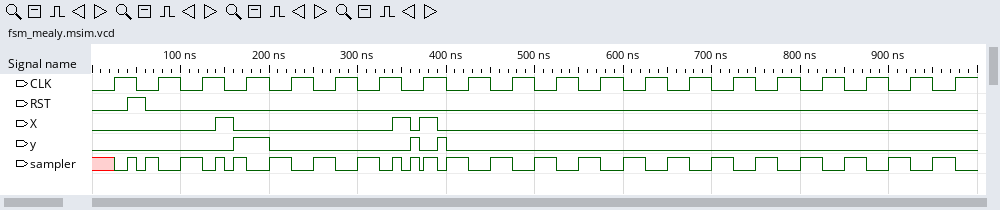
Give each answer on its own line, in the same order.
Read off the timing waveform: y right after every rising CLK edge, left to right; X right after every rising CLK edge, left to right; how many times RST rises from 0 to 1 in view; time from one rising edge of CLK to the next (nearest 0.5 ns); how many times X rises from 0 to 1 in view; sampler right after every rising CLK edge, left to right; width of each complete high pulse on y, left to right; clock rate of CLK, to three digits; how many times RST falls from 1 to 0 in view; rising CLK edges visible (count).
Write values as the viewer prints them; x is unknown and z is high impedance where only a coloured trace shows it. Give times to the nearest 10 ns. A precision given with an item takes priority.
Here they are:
0 0 0 1 0 0 0 0 0 0 0 0 0 0 0 0 0 0 0 0
0 0 0 0 0 0 0 1 0 0 0 0 0 0 0 0 0 0 0 0
1
50 ns
3
0 0 0 0 0 0 0 1 0 0 0 0 0 0 0 0 0 0 0 0
40 ns, 10 ns, 10 ns
20.0 MHz
1
20
